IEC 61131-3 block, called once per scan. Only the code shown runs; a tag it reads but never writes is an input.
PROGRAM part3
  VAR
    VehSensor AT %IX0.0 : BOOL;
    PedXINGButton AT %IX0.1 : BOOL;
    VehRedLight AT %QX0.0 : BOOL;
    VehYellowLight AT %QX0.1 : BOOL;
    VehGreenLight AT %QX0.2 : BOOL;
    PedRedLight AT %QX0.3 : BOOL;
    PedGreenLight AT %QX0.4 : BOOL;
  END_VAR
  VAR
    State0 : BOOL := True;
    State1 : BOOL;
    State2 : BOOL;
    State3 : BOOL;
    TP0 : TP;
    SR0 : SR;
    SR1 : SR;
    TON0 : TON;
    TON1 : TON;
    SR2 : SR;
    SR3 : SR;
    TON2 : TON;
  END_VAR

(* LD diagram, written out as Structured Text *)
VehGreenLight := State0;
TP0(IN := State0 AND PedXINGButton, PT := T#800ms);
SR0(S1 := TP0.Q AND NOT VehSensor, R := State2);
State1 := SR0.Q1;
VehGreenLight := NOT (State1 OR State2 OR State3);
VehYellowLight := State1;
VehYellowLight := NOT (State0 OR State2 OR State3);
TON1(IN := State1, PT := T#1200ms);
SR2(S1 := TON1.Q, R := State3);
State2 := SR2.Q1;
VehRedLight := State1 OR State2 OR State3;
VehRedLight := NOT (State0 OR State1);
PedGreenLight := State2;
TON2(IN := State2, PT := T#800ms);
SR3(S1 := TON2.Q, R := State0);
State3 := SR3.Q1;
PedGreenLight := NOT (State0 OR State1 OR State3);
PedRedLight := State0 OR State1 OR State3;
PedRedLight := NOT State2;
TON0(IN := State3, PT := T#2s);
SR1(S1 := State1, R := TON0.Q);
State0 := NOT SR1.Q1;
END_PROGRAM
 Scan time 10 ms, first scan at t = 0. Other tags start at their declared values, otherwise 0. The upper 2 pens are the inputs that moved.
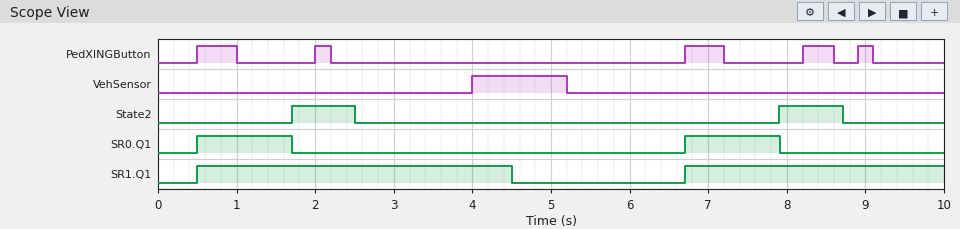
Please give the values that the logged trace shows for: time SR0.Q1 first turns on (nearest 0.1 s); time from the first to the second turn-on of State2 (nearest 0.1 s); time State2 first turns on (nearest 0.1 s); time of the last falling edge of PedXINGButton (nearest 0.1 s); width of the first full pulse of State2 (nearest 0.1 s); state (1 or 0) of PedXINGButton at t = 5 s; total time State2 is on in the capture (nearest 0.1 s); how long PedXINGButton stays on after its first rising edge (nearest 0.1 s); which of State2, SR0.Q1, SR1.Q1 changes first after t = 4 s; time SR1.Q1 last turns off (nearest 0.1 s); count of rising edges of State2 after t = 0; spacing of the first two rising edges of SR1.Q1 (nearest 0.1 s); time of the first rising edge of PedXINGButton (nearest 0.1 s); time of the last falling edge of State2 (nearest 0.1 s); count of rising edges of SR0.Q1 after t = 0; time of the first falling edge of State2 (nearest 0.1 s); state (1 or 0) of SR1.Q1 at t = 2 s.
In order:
0.5 s
6.2 s
1.7 s
9.1 s
0.8 s
0
1.6 s
0.5 s
SR1.Q1
4.5 s
2
6.2 s
0.5 s
8.7 s
2
2.5 s
1
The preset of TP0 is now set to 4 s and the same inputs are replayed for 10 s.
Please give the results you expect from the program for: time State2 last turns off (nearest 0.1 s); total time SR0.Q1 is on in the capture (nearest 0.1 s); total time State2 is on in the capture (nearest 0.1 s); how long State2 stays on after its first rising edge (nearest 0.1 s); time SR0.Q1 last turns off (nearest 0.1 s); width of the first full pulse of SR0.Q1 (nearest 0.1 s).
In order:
4.0 s
6.8 s
4.4 s
2.3 s
4.0 s
3.5 s
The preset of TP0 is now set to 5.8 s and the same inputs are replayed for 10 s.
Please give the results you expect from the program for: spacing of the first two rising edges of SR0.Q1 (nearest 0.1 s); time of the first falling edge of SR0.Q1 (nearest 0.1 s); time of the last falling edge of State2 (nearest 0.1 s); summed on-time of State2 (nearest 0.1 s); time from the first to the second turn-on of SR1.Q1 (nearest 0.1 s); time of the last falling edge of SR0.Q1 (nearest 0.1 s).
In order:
4.7 s
4.0 s
7.2 s
3.1 s
4.7 s
6.4 s
